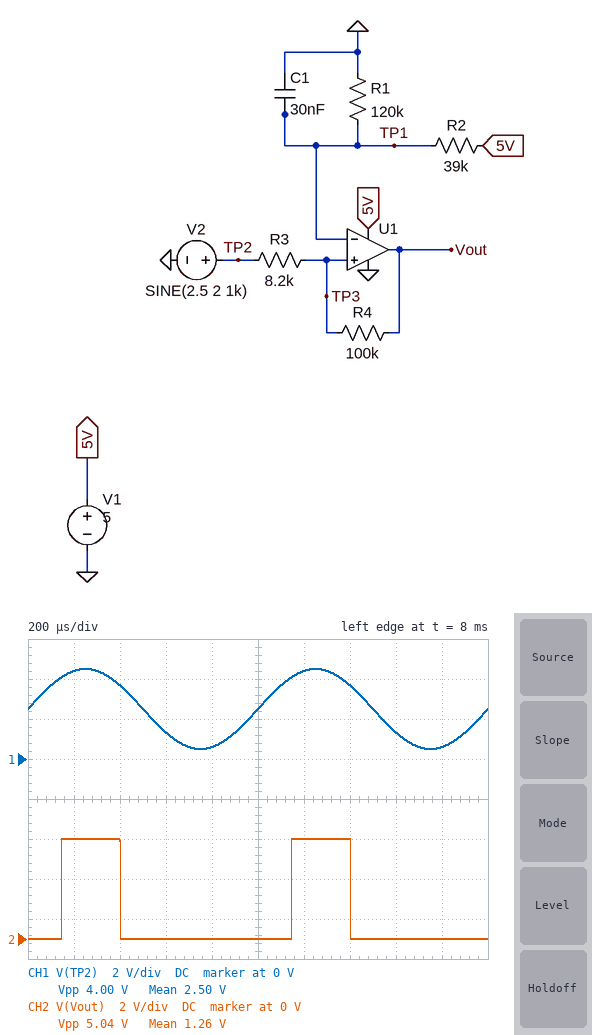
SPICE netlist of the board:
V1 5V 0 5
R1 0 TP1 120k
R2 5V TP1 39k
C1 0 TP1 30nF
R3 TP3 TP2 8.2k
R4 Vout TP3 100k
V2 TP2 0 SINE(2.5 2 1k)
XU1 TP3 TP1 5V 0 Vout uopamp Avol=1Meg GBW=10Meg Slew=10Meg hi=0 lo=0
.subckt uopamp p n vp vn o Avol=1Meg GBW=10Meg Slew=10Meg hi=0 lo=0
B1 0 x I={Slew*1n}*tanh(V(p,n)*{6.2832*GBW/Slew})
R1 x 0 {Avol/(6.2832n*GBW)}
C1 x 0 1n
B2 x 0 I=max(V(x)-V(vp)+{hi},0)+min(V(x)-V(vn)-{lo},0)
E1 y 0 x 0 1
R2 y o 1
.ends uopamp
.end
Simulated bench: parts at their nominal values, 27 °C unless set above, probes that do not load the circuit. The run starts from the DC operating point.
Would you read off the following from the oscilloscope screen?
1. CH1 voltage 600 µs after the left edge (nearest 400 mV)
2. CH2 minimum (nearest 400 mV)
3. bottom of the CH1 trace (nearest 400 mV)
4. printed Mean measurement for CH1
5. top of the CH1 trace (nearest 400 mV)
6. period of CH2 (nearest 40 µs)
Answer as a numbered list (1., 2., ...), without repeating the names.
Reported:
1. 1.2 V
2. 0 V
3. 400 mV
4. 2.50 V
5. 4.4 V
6. 1.00 ms
